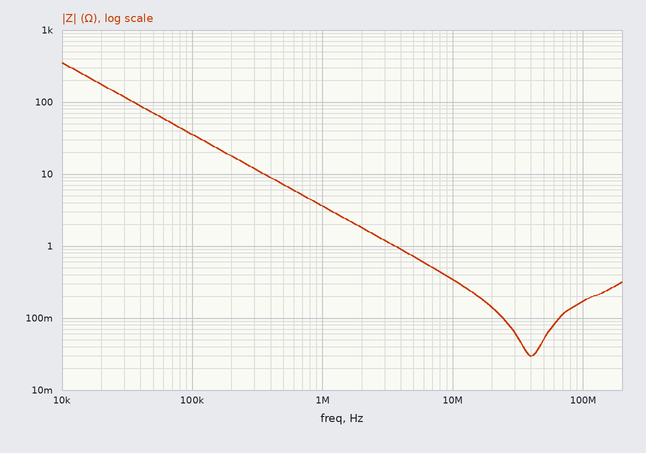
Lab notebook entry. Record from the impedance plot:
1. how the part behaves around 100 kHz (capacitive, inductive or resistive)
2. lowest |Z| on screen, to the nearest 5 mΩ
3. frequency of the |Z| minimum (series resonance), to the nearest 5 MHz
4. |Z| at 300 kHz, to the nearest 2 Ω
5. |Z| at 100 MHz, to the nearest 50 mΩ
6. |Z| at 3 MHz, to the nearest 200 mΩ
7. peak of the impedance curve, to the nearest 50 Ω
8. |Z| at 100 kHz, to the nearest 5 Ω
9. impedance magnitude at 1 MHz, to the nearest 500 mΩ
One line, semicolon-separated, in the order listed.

capacitive; 30 mΩ; 40 MHz; 12 Ω; 150 mΩ; 1.2 Ω; 350 Ω; 35 Ω; 3.5 Ω
